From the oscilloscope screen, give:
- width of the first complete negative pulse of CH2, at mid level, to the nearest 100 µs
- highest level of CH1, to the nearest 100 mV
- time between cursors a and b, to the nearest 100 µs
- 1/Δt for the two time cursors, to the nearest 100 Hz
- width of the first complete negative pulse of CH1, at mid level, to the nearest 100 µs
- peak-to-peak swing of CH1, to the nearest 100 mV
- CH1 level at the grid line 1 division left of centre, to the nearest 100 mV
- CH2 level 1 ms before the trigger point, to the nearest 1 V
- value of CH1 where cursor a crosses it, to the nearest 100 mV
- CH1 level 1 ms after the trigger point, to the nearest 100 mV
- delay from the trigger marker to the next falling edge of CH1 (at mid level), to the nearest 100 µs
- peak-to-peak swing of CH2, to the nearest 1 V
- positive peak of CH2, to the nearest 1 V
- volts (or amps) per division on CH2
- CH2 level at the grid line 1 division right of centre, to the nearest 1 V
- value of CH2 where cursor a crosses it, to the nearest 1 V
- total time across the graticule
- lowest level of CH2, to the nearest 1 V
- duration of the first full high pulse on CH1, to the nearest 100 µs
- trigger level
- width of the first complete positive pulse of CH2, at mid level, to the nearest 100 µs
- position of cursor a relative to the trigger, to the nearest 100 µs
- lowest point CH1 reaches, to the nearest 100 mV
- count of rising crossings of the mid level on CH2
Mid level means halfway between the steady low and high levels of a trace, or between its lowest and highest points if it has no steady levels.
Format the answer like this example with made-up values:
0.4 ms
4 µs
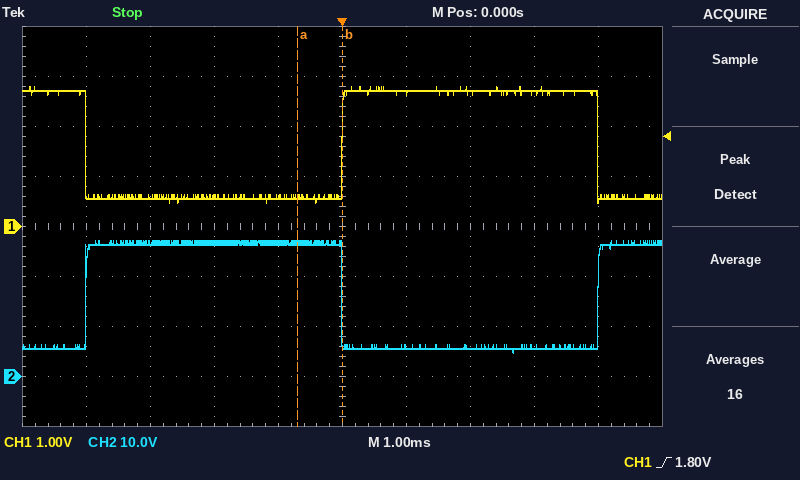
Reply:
4.0 ms
2.8 V
700 µs
1.4 kHz
4.0 ms
2.3 V
600 mV
27 V
600 mV
2.7 V
4.0 ms
22 V
27 V
10 V
6 V
27 V
10 ms
5 V
4.0 ms
1.80 V
4.0 ms
-700 µs
500 mV
2
